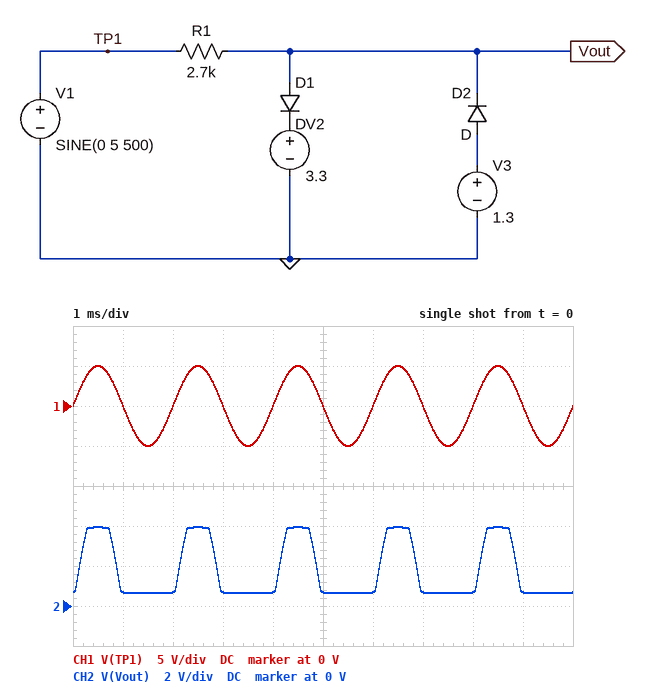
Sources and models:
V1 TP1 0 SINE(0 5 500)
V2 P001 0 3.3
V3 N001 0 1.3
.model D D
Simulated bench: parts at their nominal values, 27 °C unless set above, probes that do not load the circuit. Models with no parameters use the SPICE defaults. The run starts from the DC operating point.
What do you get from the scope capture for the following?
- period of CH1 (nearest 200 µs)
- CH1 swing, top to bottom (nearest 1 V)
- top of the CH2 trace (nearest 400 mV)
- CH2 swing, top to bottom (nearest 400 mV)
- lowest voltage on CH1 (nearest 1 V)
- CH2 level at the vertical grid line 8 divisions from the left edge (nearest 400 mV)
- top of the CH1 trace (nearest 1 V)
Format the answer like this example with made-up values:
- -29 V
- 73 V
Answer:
- 2.0 ms
- 10 V
- 4.0 V
- 3.2 V
- -5 V
- 800 mV
- 5 V
